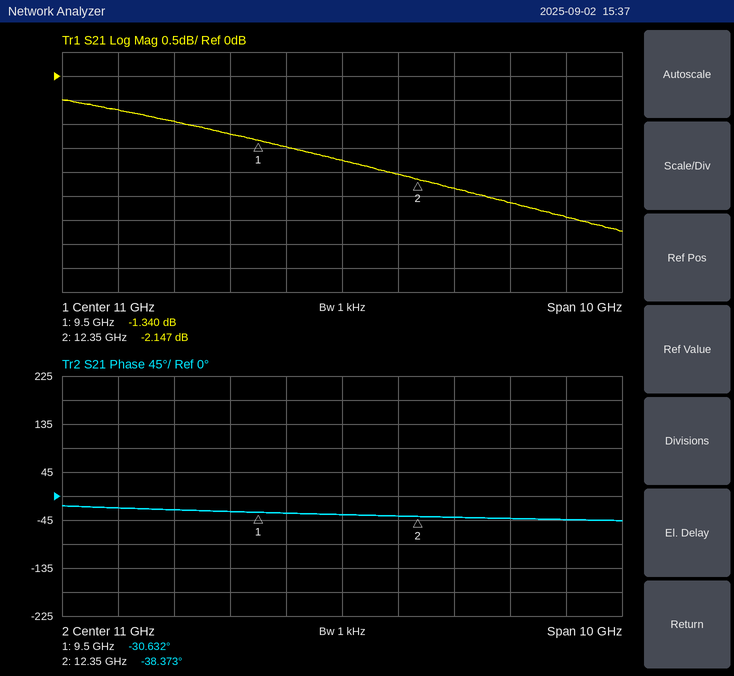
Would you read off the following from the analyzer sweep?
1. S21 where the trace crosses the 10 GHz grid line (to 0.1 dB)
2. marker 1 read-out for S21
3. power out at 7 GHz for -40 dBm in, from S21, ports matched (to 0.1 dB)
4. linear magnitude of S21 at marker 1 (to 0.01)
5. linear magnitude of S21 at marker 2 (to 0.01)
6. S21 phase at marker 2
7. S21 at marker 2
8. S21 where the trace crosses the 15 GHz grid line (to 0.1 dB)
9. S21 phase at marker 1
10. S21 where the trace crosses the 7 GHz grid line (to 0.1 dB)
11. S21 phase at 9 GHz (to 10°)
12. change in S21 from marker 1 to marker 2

-1.5 dB
-1.340 dB
-40.7 dBm
0.86
0.78
-38.373°
-2.147 dB
-2.9 dB
-30.632°
-0.7 dB
-30°
-0.807 dB
